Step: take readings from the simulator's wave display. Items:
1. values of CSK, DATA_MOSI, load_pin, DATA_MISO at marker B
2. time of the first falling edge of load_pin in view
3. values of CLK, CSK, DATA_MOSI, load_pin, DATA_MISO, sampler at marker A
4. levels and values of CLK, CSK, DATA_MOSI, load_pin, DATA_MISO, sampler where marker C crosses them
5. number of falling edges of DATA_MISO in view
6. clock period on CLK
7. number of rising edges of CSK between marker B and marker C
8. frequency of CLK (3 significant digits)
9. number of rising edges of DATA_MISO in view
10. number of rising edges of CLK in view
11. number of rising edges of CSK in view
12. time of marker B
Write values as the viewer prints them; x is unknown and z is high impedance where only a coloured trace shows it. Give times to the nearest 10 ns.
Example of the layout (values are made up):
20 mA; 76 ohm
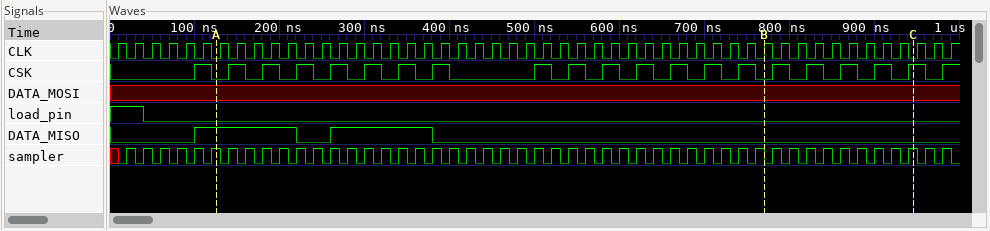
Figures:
CSK=0, DATA_MOSI=x, load_pin=0, DATA_MISO=0; 40 ns; CLK=0, CSK=0, DATA_MOSI=x, load_pin=0, DATA_MISO=1, sampler=1; CLK=0, CSK=1, DATA_MOSI=x, load_pin=0, DATA_MISO=0, sampler=1; 2; 20 ns; 5; 50.0 MHz; 2; 50; 21; 770 ns
